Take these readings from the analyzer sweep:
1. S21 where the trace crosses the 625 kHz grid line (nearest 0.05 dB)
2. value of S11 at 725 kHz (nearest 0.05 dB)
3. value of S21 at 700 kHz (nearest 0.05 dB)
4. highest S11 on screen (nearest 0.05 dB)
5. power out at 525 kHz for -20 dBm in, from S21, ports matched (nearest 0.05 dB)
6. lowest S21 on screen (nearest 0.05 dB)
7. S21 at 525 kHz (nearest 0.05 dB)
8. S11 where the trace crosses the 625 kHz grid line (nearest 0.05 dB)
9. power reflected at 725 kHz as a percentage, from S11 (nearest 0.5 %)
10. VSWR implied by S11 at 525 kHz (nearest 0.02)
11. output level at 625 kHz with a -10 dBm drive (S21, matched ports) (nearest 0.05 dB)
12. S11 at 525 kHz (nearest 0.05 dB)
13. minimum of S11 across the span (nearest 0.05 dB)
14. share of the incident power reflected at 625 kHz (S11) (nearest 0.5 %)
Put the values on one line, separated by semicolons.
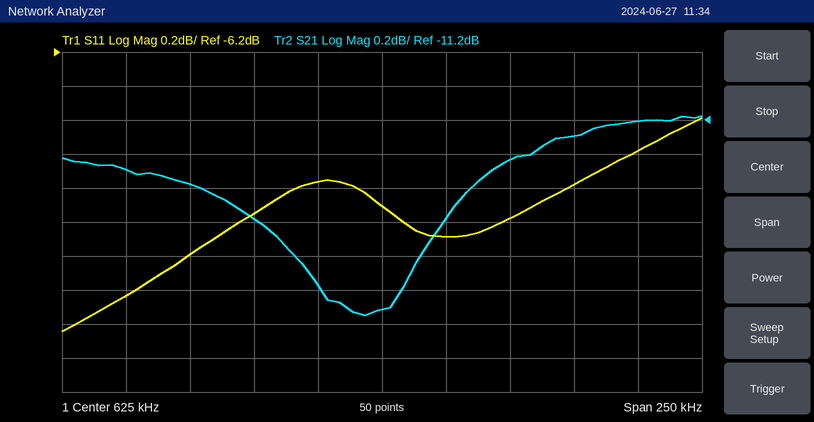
-12.30 dB; -6.80 dB; -11.30 dB; -6.60 dB; -31.50 dBm; -12.35 dB; -11.50 dB; -7.10 dB; 21.0 %; 2.42; -22.30 dBm; -7.65 dB; -7.85 dB; 19.5 %
